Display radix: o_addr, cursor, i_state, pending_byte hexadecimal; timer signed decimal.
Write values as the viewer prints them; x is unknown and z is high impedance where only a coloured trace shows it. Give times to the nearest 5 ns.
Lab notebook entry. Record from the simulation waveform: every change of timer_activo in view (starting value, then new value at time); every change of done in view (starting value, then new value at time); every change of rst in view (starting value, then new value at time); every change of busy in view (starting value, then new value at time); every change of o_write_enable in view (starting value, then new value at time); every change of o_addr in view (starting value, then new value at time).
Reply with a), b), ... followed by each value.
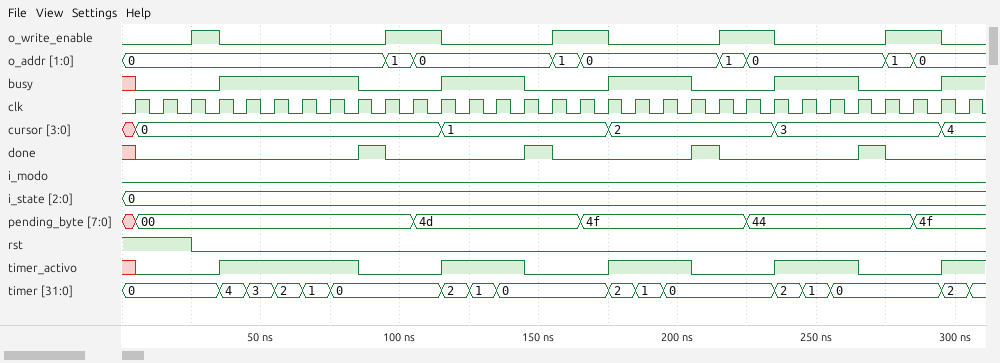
a) x, 0 at 5 ns, 1 at 35 ns, 0 at 85 ns, 1 at 115 ns, 0 at 145 ns, 1 at 175 ns, 0 at 205 ns, 1 at 235 ns, 0 at 265 ns, 1 at 295 ns
b) x, 0 at 5 ns, 1 at 85 ns, 0 at 95 ns, 1 at 145 ns, 0 at 155 ns, 1 at 205 ns, 0 at 215 ns, 1 at 265 ns, 0 at 275 ns
c) 1, 0 at 25 ns
d) x, 0 at 5 ns, 1 at 35 ns, 0 at 85 ns, 1 at 115 ns, 0 at 145 ns, 1 at 175 ns, 0 at 205 ns, 1 at 235 ns, 0 at 265 ns, 1 at 295 ns
e) 0, 1 at 25 ns, 0 at 35 ns, 1 at 95 ns, 0 at 115 ns, 1 at 155 ns, 0 at 175 ns, 1 at 215 ns, 0 at 235 ns, 1 at 275 ns, 0 at 295 ns
f) 0, 1 at 95 ns, 0 at 105 ns, 1 at 155 ns, 0 at 165 ns, 1 at 215 ns, 0 at 225 ns, 1 at 275 ns, 0 at 285 ns
